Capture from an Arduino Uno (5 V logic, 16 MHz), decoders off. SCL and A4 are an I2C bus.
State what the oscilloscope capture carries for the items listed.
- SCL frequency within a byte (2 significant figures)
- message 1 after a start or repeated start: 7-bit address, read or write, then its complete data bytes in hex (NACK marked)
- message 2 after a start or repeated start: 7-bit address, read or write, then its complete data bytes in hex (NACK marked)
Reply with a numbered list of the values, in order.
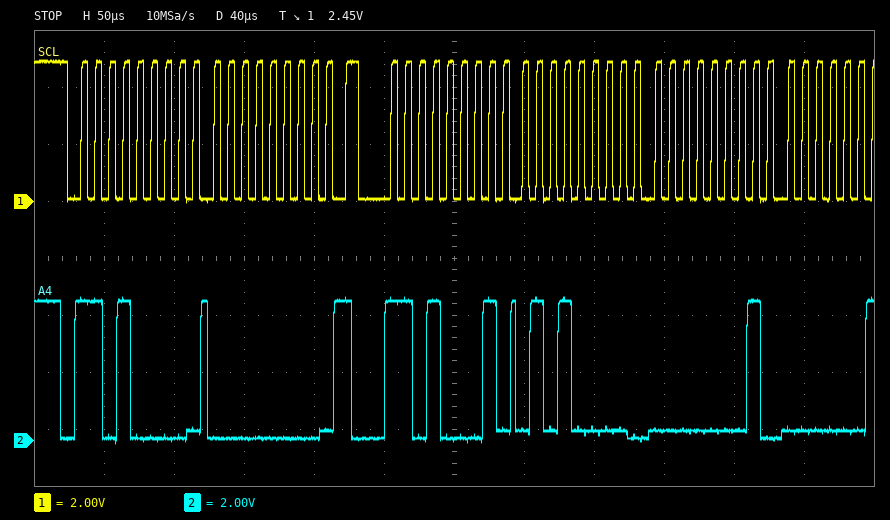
1. 100 kHz
2. 0x68 write: 00
3. 0x68 read: 50 01
